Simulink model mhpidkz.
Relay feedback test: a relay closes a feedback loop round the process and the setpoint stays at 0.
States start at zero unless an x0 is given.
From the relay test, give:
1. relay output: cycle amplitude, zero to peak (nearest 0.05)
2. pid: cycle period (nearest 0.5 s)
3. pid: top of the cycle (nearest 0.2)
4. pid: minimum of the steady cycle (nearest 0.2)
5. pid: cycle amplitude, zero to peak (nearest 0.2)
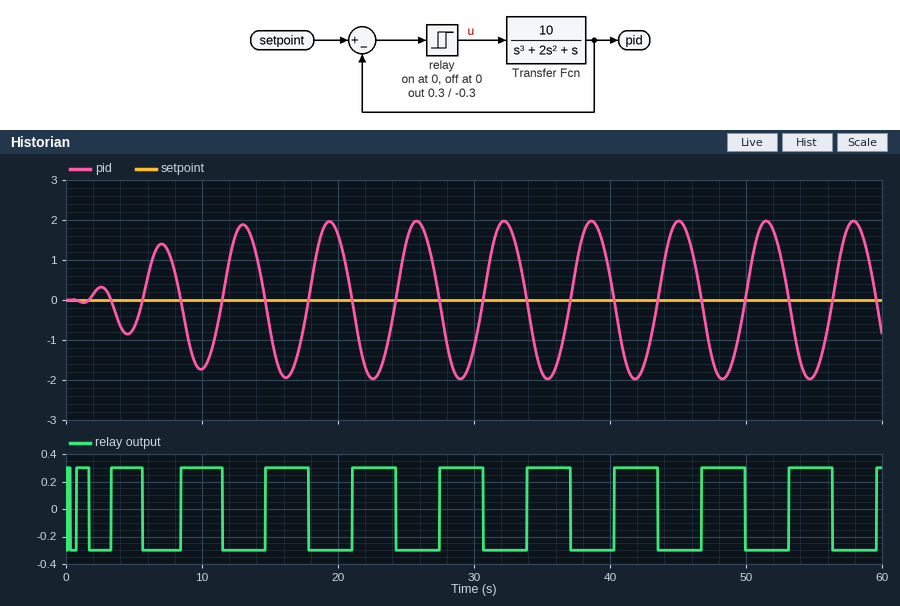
0.30
6.5 s
2.0
-2.0
2.0
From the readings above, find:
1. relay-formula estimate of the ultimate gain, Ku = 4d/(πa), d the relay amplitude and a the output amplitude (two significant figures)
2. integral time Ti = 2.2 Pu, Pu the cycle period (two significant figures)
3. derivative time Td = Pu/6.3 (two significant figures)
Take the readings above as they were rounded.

0.19
14 s
1.0 s
